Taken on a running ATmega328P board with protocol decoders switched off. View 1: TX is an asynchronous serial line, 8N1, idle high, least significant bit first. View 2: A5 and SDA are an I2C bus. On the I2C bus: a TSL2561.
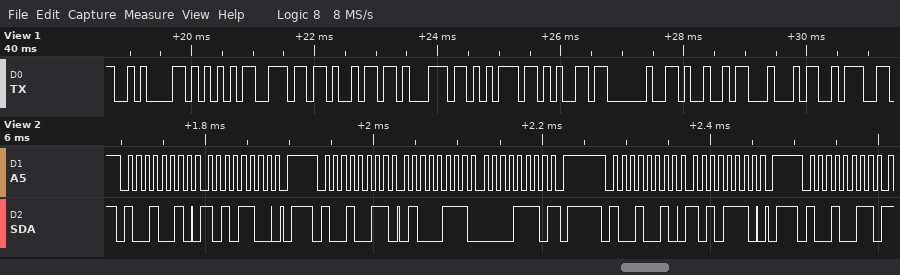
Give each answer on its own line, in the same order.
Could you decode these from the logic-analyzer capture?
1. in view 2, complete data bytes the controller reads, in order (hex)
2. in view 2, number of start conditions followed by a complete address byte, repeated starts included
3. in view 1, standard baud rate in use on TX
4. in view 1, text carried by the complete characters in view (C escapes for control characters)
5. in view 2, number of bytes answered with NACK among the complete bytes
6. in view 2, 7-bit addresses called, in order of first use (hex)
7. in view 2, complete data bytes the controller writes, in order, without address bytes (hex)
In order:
47 0E
4
9600 baud
"\nUnique ID:"
1
0x49
AC AE
